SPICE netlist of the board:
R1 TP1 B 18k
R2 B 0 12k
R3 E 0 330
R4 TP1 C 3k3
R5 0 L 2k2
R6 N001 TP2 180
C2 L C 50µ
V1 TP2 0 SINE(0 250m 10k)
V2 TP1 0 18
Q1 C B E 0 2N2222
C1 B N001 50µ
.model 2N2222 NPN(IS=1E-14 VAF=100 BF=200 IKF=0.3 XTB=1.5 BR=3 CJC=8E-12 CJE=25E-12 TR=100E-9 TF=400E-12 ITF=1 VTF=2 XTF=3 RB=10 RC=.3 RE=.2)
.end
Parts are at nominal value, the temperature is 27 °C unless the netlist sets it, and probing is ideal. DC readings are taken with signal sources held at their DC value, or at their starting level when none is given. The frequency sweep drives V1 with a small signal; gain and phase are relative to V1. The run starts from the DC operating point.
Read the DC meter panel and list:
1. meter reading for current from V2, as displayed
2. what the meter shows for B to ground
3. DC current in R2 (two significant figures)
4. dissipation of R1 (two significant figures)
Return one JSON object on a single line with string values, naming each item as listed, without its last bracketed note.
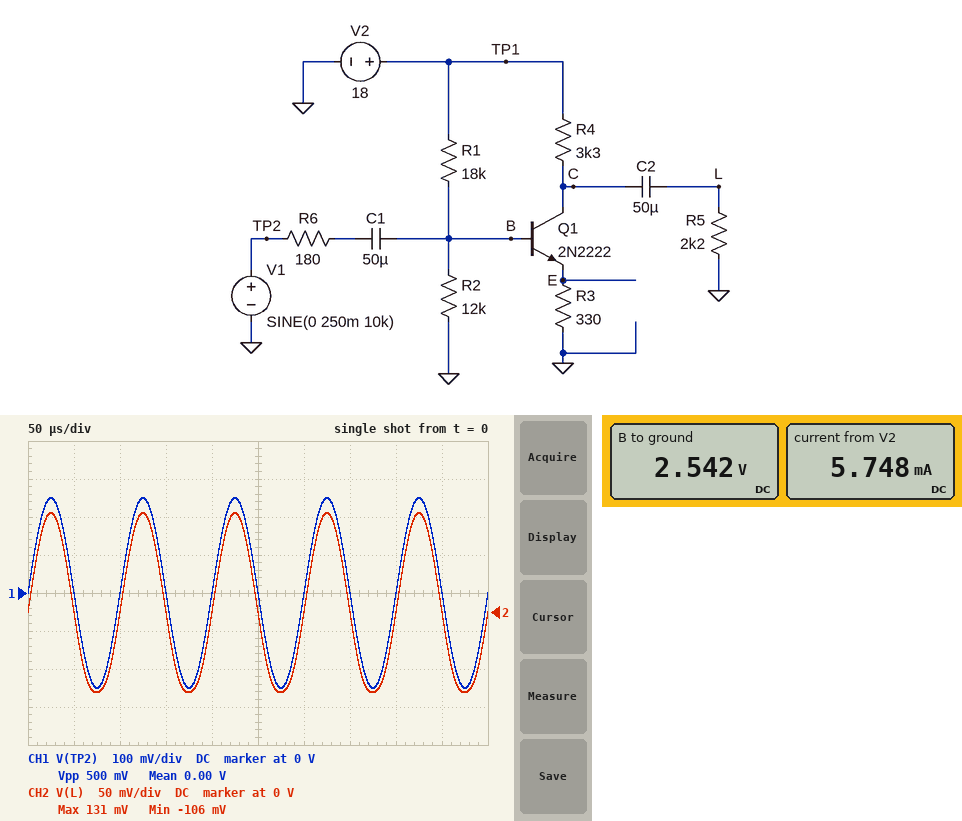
{"meter reading for current from V2, as displayed": "5.748 mA", "what the meter shows for B to ground": "2.542 V", "DC current in R2": "210 µA", "dissipation of R1": "13 mW"}
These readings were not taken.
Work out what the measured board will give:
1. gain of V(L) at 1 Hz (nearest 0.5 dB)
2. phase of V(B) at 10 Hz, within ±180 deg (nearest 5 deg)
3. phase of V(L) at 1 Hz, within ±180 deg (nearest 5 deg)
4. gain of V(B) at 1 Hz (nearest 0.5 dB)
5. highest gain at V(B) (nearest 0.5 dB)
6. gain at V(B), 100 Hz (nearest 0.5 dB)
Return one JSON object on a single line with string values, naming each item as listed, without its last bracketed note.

{"gain of V(L) at 1 Hz": "-27.0 dB", "phase of V(B) at 10 Hz, within ±180 deg": "35 deg", "phase of V(L) at 1 Hz, within ±180 deg": "135 deg", "gain of V(B) at 1 Hz": "-20.5 dB", "highest gain at V(B)": "-4.5 dB", "gain at V(B), 100 Hz": "-4.5 dB"}
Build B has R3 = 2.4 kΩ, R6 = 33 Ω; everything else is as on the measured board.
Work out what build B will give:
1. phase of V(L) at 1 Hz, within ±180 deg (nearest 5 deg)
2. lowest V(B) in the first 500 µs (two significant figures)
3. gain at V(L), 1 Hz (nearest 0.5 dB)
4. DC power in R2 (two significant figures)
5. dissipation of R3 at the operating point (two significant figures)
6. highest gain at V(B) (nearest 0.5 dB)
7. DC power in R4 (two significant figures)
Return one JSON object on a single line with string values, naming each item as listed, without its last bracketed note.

{"phase of V(L) at 1 Hz, within ±180 deg": "-125 deg", "lowest V(B) in the first 500 µs": "6.9 V", "gain at V(L), 1 Hz": "-7.5 dB", "DC power in R2": "4.2 mW", "dissipation of R3 at the operating point": "17 mW", "highest gain at V(B)": "0 dB", "DC power in R4": "23 mW"}
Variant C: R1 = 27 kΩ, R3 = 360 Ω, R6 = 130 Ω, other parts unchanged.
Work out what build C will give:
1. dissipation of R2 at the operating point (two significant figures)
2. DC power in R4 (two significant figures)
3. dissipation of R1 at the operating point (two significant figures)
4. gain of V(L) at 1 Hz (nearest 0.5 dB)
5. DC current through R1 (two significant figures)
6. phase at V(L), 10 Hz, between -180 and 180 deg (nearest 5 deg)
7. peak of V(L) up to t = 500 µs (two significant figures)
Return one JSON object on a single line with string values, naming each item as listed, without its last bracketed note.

{"dissipation of R2 at the operating point": "560 µW", "DC power in R4": "78 mW", "dissipation of R1 at the operating point": "8.8 mW", "gain of V(L) at 1 Hz": "-27.5 dB", "DC current through R1": "570 µA", "phase at V(L), 10 Hz, between -180 and 180 deg": "45 deg", "peak of V(L) up to t = 500 µs": "270 mV"}
